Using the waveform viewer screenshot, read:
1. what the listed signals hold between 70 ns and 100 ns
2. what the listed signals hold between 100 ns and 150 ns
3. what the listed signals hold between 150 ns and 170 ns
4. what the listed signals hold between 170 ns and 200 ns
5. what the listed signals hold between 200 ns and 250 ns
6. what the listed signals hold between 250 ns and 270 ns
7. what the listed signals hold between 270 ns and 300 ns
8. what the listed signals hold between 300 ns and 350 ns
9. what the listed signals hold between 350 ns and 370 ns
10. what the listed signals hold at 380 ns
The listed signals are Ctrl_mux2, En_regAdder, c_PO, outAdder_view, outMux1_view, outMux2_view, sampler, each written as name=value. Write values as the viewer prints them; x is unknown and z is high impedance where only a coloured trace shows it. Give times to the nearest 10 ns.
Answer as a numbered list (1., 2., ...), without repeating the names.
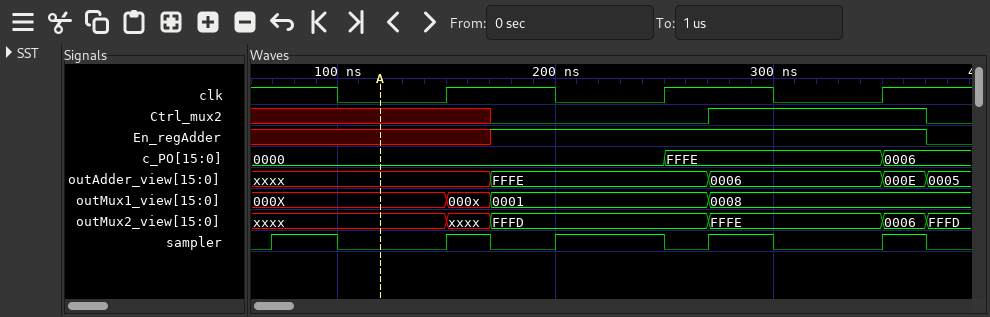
1. Ctrl_mux2=x, En_regAdder=x, c_PO=0000, outAdder_view=xxxx, outMux1_view=000X, outMux2_view=xxxx, sampler=1
2. Ctrl_mux2=x, En_regAdder=x, c_PO=0000, outAdder_view=xxxx, outMux1_view=000X, outMux2_view=xxxx, sampler=0
3. Ctrl_mux2=x, En_regAdder=x, c_PO=0000, outAdder_view=xxxx, outMux1_view=000x, outMux2_view=xxxx, sampler=1
4. Ctrl_mux2=0, En_regAdder=1, c_PO=0000, outAdder_view=FFFE, outMux1_view=0001, outMux2_view=FFFD, sampler=0
5. Ctrl_mux2=0, En_regAdder=1, c_PO=0000, outAdder_view=FFFE, outMux1_view=0001, outMux2_view=FFFD, sampler=1
6. Ctrl_mux2=0, En_regAdder=1, c_PO=FFFE, outAdder_view=FFFE, outMux1_view=0001, outMux2_view=FFFD, sampler=0
7. Ctrl_mux2=1, En_regAdder=1, c_PO=FFFE, outAdder_view=0006, outMux1_view=0008, outMux2_view=FFFE, sampler=1
8. Ctrl_mux2=1, En_regAdder=1, c_PO=FFFE, outAdder_view=0006, outMux1_view=0008, outMux2_view=FFFE, sampler=0
9. Ctrl_mux2=1, En_regAdder=1, c_PO=0006, outAdder_view=000E, outMux1_view=0008, outMux2_view=0006, sampler=1
10. Ctrl_mux2=0, En_regAdder=0, c_PO=0006, outAdder_view=0005, outMux1_view=0008, outMux2_view=FFFD, sampler=0
